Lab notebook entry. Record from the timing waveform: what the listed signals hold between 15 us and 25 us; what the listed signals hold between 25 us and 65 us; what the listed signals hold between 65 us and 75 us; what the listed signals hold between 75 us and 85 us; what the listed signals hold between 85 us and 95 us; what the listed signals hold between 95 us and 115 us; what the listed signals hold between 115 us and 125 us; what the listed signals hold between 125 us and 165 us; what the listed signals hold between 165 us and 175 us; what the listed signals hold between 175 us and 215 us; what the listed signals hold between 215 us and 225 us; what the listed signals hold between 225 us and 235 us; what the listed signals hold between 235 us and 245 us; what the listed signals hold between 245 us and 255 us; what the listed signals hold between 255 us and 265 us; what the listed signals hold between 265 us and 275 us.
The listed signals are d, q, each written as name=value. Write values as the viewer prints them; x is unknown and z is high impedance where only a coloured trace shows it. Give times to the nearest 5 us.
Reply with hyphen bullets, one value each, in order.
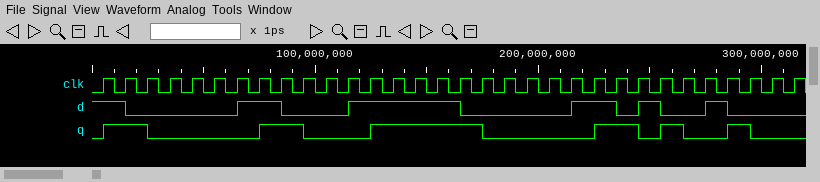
- d=0, q=1
- d=0, q=0
- d=1, q=0
- d=1, q=1
- d=0, q=1
- d=0, q=0
- d=1, q=0
- d=1, q=1
- d=0, q=1
- d=0, q=0
- d=1, q=0
- d=1, q=1
- d=0, q=1
- d=1, q=0
- d=0, q=1
- d=0, q=0
